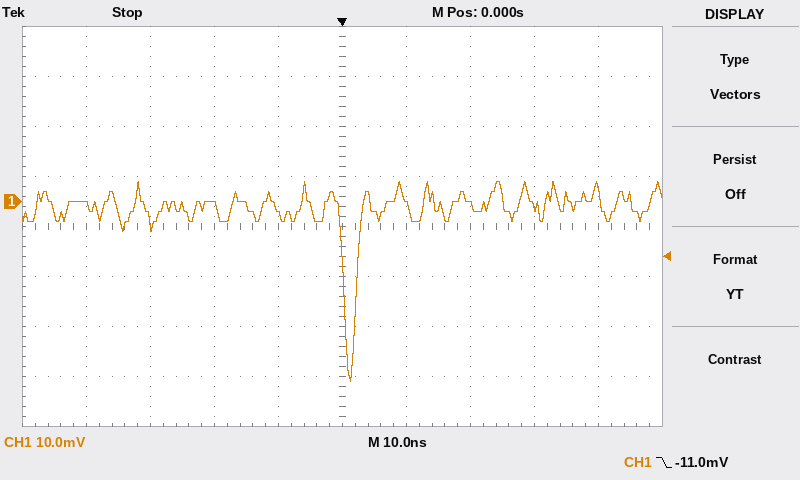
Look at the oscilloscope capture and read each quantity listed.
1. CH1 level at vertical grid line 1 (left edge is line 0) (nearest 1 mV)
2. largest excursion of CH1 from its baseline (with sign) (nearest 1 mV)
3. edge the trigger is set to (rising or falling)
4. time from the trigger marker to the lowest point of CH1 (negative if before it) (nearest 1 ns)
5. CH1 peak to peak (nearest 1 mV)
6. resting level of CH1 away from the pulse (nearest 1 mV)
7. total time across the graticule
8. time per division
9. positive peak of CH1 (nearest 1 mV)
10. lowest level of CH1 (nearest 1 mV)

-1 mV
-35 mV
falling
+1 ns
40 mV
-1 mV
100 ns
10 ns
4 mV
-36 mV
